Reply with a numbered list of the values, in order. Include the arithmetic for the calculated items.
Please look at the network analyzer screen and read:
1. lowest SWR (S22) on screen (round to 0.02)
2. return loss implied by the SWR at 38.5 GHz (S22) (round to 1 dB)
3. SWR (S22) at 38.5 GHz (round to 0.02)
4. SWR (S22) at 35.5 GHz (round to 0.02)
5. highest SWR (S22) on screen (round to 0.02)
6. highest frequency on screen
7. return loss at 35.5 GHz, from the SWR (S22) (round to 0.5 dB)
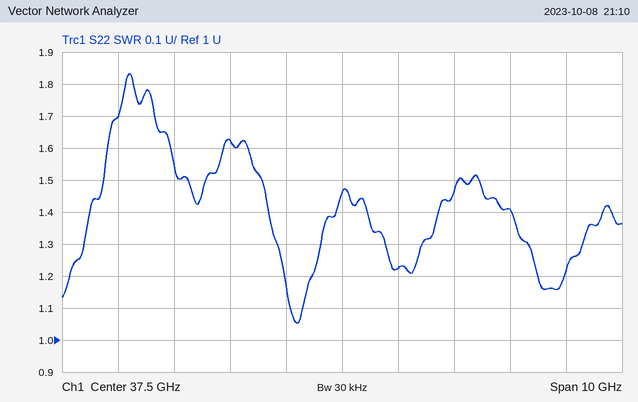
1. 1.06
2. −20 log10((1.22 − 1)/(1.22 + 1)) ≈ 20 dB
3. 1.22
4. 1.62
5. 1.84
6. 42.5 GHz
7. −20 log10((1.62 − 1)/(1.62 + 1)) ≈ 12.5 dB
